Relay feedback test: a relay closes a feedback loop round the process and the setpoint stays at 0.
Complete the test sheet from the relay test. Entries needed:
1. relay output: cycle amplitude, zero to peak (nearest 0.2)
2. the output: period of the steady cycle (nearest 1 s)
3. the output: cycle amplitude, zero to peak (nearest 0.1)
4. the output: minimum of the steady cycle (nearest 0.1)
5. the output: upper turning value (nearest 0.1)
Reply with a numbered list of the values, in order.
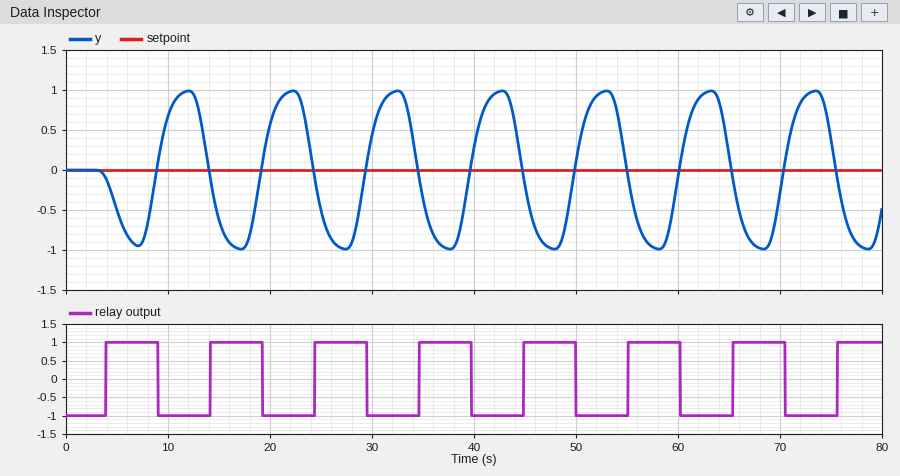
1. 1.0
2. 10 s
3. 1.0
4. -1.0
5. 1.0
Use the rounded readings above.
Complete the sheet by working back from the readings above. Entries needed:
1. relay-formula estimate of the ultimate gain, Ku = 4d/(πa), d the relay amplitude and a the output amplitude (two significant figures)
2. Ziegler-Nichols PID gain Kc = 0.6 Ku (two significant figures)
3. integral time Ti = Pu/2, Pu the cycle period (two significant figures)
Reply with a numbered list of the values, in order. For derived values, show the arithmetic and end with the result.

1. 4 × 1 / (π × 1) = 1.3
2. 0.6 × 1.3 = 0.78
3. 10 / 2 = 5.0 s
